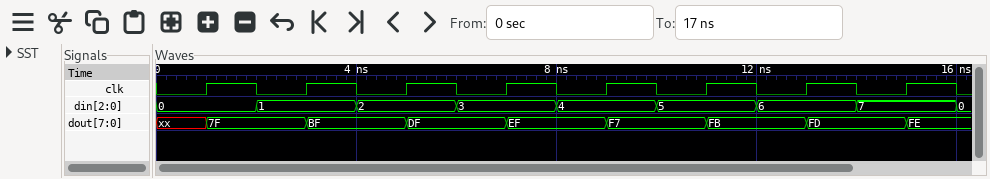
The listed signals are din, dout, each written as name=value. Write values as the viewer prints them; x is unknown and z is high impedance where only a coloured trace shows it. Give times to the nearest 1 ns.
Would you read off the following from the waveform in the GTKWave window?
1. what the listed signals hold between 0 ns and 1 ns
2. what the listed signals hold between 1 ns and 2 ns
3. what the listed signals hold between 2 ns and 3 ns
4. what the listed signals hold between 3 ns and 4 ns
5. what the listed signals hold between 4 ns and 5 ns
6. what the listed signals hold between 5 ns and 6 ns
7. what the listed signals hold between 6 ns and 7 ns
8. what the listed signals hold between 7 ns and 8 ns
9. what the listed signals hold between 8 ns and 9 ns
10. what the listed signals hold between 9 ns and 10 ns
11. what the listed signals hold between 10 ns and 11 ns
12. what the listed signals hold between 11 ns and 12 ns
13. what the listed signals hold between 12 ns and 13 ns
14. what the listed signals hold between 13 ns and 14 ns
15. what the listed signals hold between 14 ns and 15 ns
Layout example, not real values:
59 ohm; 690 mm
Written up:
din=0, dout=xx; din=0, dout=7F; din=1, dout=7F; din=1, dout=BF; din=2, dout=BF; din=2, dout=DF; din=3, dout=DF; din=3, dout=EF; din=4, dout=EF; din=4, dout=F7; din=5, dout=F7; din=5, dout=FB; din=6, dout=FB; din=6, dout=FD; din=7, dout=FD
